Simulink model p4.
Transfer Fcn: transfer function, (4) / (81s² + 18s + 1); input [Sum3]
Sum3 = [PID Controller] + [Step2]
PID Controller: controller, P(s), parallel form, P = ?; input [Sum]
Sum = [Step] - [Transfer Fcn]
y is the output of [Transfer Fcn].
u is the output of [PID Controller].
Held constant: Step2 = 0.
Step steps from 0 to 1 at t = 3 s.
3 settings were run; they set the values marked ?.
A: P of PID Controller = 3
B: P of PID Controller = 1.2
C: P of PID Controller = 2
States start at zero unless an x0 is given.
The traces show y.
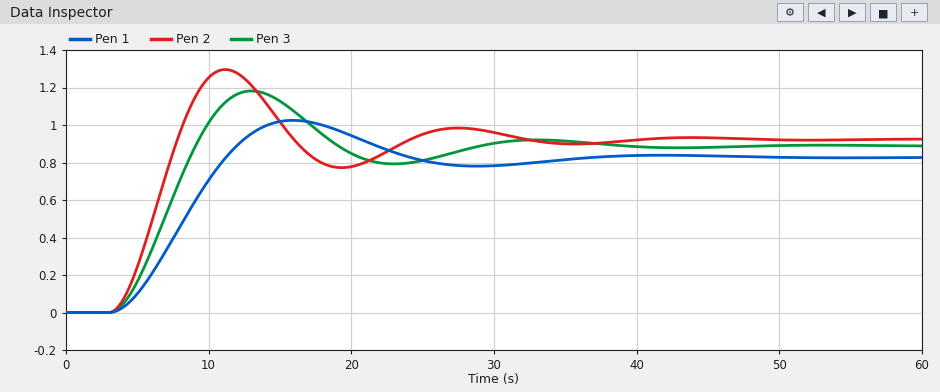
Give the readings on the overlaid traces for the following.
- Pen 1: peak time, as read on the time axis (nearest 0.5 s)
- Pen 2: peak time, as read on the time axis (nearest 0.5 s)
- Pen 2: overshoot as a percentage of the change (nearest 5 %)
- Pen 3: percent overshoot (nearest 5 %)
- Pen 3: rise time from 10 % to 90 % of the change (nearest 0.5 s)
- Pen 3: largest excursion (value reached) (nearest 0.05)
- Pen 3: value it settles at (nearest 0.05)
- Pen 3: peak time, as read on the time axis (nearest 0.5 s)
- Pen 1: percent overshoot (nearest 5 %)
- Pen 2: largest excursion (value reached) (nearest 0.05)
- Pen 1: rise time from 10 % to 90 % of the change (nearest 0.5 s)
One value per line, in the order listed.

16.0 s
11.0 s
40 %
35 %
4.0 s
1.20
0.90
13.0 s
25 %
1.30
5.5 s
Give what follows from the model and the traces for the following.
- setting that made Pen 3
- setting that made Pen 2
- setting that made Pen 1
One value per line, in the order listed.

C
A
B
